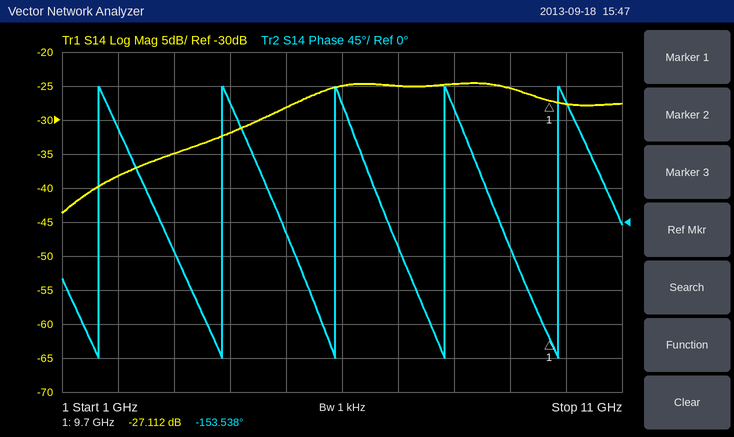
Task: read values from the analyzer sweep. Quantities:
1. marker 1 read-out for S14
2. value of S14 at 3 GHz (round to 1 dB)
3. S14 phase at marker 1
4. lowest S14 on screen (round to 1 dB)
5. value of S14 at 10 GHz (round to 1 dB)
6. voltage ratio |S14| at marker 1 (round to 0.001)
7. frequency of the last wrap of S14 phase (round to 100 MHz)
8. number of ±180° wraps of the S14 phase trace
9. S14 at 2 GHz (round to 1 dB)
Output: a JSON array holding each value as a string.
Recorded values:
["-27.112 dB", "-35 dB", "-153.538°", "-44 dB", "-28 dB", "0.044", "9.9 GHz", "5", "-38 dB"]
